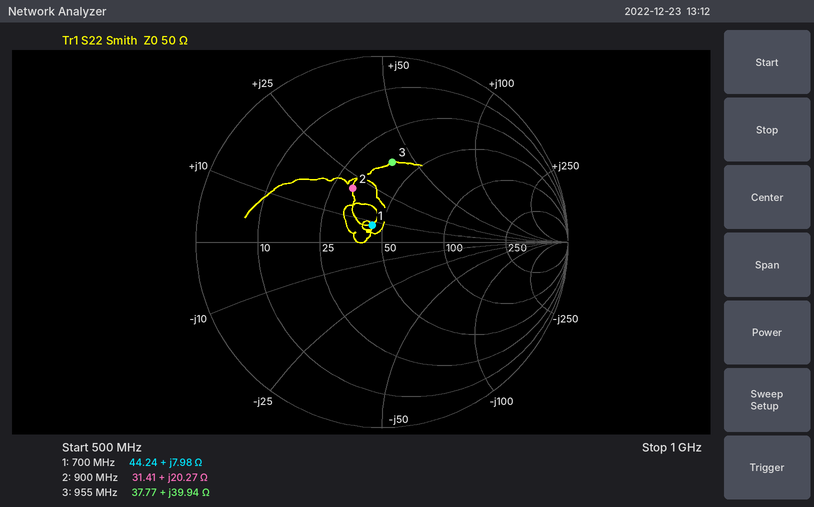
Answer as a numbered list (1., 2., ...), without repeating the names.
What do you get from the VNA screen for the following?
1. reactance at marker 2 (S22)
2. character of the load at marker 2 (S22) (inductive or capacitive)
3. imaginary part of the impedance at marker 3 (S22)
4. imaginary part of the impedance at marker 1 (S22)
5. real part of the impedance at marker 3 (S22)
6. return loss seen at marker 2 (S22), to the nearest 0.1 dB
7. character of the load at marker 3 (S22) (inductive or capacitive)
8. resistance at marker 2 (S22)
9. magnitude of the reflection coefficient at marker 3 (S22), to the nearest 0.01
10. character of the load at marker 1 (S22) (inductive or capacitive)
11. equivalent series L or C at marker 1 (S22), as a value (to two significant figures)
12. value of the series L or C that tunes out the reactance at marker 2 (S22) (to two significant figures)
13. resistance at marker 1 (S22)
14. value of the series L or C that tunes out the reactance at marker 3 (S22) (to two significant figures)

1. +20.27 Ω
2. inductive
3. +39.94 Ω
4. +7.98 Ω
5. 37.77 Ω
6. 9.7 dB
7. inductive
8. 31.41 Ω
9. 0.43
10. inductive
11. 1.8 nH
12. 8.7 pF
13. 44.24 Ω
14. 4.2 pF
